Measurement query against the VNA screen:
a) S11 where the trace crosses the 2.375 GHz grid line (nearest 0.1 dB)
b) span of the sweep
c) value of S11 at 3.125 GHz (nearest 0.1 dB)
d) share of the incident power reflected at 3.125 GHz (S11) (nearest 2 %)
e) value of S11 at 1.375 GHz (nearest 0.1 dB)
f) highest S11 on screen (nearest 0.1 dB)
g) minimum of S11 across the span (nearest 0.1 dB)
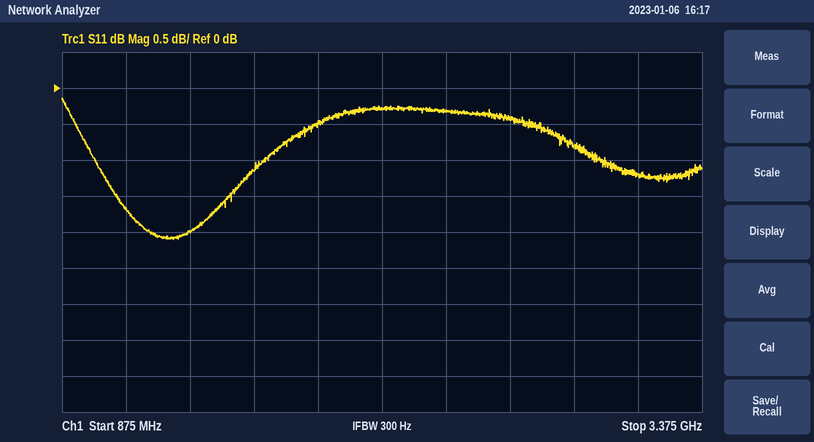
-0.3 dB
2.5 GHz
-1.2 dB
76 %
-2.0 dB
-0.1 dB
-2.1 dB
